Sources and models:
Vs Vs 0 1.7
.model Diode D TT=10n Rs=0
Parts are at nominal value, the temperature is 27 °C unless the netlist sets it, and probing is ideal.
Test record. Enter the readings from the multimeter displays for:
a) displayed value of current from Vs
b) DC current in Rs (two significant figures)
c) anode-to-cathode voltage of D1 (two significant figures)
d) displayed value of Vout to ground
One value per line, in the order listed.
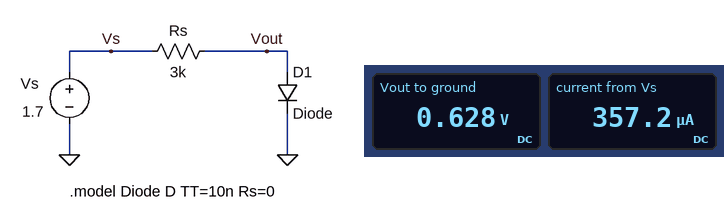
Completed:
357.2 µA
360 µA
630 mV
0.628 V
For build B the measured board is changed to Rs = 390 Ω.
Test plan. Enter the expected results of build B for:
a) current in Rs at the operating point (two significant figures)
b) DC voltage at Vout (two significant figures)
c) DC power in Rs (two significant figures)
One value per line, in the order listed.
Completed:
2.6 mA
680 mV
2.7 mW
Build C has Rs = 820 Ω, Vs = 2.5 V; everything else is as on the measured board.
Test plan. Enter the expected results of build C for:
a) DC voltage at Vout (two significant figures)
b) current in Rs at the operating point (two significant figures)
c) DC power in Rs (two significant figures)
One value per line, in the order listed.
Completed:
680 mV
2.2 mA
4.1 mW
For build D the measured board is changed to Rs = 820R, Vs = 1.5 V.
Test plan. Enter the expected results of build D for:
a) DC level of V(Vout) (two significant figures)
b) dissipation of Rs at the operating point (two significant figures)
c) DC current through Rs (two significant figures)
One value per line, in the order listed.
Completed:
660 mV
870 µW
1.0 mA
